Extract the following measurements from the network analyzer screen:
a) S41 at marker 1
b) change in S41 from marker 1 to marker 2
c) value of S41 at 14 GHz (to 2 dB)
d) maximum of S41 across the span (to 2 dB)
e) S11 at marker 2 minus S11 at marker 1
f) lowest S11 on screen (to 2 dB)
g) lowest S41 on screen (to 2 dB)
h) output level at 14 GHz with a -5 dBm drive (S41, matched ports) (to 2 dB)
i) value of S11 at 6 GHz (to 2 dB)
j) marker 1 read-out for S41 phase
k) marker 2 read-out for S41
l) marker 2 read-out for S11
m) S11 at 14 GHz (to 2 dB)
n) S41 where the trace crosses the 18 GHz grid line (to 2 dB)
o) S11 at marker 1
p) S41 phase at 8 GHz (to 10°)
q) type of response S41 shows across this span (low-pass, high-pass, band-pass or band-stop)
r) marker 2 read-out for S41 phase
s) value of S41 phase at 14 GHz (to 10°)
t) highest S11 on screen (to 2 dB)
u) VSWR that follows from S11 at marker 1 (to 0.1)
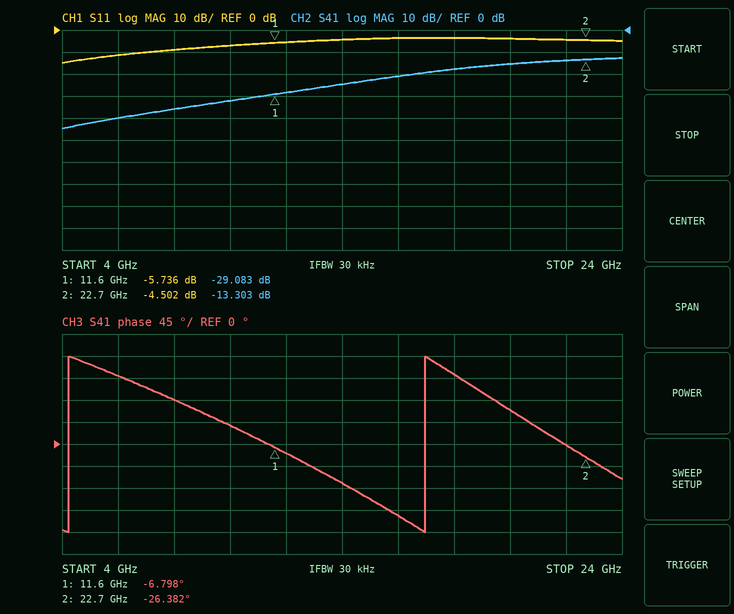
-29.083 dB
15.780 dB
-24 dB
-12 dB
1.234 dB
-14 dB
-44 dB
-30 dBm
-12 dB
-6.798°
-13.303 dB
-4.502 dB
-4 dB
-18 dB
-5.736 dB
90°
high-pass
-26.382°
-80°
-4 dB
3.1
